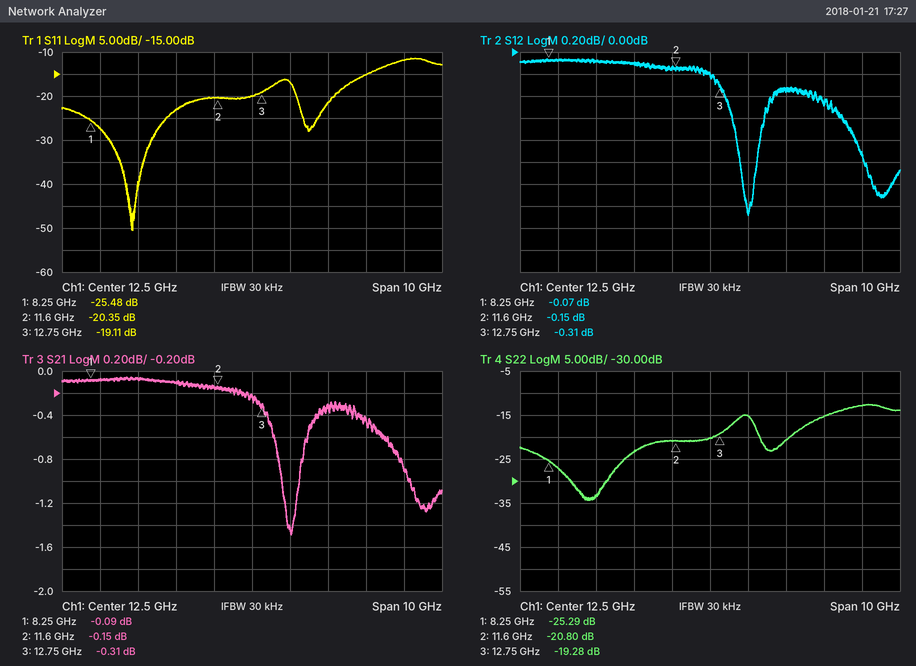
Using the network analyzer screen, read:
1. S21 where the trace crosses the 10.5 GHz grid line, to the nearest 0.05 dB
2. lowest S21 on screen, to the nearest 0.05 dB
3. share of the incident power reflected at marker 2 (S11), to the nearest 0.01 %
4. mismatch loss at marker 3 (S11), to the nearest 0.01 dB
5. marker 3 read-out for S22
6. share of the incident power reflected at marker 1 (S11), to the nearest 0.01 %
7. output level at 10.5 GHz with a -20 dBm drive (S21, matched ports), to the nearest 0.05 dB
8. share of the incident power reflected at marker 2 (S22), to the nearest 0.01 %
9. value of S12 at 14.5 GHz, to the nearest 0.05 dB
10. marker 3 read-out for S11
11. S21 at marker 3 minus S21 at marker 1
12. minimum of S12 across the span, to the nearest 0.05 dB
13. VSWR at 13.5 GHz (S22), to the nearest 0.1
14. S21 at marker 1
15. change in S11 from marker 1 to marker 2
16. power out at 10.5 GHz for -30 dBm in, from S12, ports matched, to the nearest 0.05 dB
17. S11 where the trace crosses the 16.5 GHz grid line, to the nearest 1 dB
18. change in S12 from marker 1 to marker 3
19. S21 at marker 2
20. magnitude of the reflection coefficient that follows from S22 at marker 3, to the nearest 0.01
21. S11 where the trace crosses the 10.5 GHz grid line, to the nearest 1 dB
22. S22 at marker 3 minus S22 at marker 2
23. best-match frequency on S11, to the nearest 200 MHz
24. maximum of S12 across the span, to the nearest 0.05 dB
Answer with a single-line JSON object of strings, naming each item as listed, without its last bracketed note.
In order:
{"S21 where the trace crosses the 10.5 GHz grid line, to the nearest 0.05 dB": "-0.10 dB", "lowest S21 on screen, to the nearest 0.05 dB": "-1.50 dB", "share of the incident power reflected at marker 2 (S11), to the nearest 0.01 %": "0.92 %", "mismatch loss at marker 3 (S11), to the nearest 0.01 dB": "0.05 dB", "marker 3 read-out for S22": "-19.28 dB", "share of the incident power reflected at marker 1 (S11), to the nearest 0.01 %": "0.28 %", "output level at 10.5 GHz with a -20 dBm drive (S21, matched ports), to the nearest 0.05 dB": "-20.10 dBm", "share of the incident power reflected at marker 2 (S22), to the nearest 0.01 %": "0.83 %", "value of S12 at 14.5 GHz, to the nearest 0.05 dB": "-0.35 dB", "marker 3 read-out for S11": "-19.11 dB", "S21 at marker 3 minus S21 at marker 1": "-0.22 dB", "minimum of S12 across the span, to the nearest 0.05 dB": "-1.50 dB", "VSWR at 13.5 GHz (S22), to the nearest 0.1": "1.4", "S21 at marker 1": "-0.09 dB", "change in S11 from marker 1 to marker 2": "5.13 dB", "power out at 10.5 GHz for -30 dBm in, from S12, ports matched, to the nearest 0.05 dB": "-30.10 dBm", "S11 where the trace crosses the 16.5 GHz grid line, to the nearest 1 dB": "-12 dB", "change in S12 from marker 1 to marker 3": "-0.24 dB", "S21 at marker 2": "-0.15 dB", "magnitude of the reflection coefficient that follows from S22 at marker 3, to the nearest 0.01": "0.11", "S11 where the trace crosses the 10.5 GHz grid line, to the nearest 1 dB": "-23 dB", "S22 at marker 3 minus S22 at marker 2": "1.52 dB", "best-match frequency on S11, to the nearest 200 MHz": "9.4 GHz", "maximum of S12 across the span, to the nearest 0.05 dB": "-0.05 dB"}
